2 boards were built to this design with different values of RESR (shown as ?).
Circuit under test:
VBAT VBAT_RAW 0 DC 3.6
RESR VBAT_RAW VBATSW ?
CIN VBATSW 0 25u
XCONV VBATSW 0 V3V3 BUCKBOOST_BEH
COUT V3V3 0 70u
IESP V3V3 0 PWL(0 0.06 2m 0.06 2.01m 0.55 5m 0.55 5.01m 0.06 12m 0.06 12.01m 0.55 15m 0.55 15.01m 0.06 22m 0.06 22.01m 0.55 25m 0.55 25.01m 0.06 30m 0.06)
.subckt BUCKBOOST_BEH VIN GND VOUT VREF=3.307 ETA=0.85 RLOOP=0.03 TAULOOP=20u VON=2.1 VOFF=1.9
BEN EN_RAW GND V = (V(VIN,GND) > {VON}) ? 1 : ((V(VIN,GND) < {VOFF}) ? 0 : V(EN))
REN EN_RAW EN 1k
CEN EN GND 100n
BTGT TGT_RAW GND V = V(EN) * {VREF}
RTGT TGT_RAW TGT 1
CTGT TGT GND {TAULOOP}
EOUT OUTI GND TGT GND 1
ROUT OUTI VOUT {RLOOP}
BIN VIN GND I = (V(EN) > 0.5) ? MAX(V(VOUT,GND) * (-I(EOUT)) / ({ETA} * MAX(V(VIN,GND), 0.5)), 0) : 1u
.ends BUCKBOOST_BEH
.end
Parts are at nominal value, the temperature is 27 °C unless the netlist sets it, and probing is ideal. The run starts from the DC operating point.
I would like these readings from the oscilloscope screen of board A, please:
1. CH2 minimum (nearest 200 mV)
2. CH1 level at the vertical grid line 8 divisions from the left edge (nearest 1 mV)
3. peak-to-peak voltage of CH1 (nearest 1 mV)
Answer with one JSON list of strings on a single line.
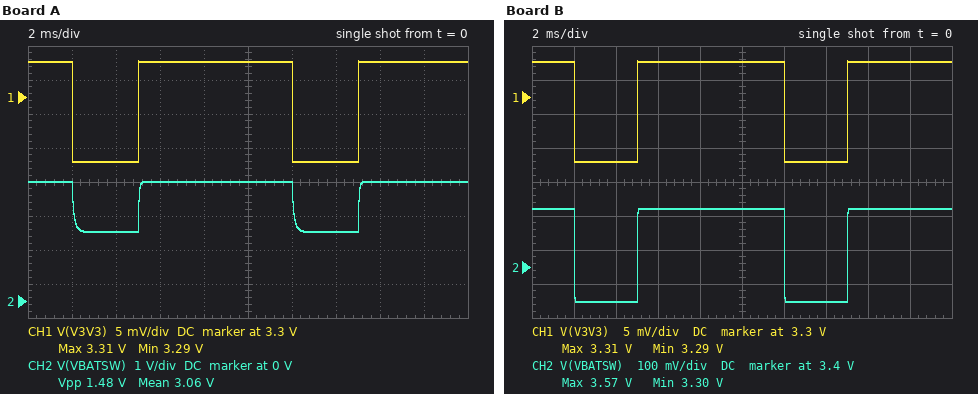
["2.0 V", "3.305 V", "15 mV"]
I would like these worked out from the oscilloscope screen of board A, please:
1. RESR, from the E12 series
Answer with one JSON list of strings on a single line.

["1.5 Ω"]
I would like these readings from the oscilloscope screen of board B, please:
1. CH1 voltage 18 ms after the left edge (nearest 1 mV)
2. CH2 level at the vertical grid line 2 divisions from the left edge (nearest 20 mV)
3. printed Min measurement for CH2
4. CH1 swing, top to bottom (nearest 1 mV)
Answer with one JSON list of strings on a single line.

["3.305 V", "3.30 V", "3.30 V", "15 mV"]
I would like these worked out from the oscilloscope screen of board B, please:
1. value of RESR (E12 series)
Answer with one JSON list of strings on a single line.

["0.47 Ω"]
